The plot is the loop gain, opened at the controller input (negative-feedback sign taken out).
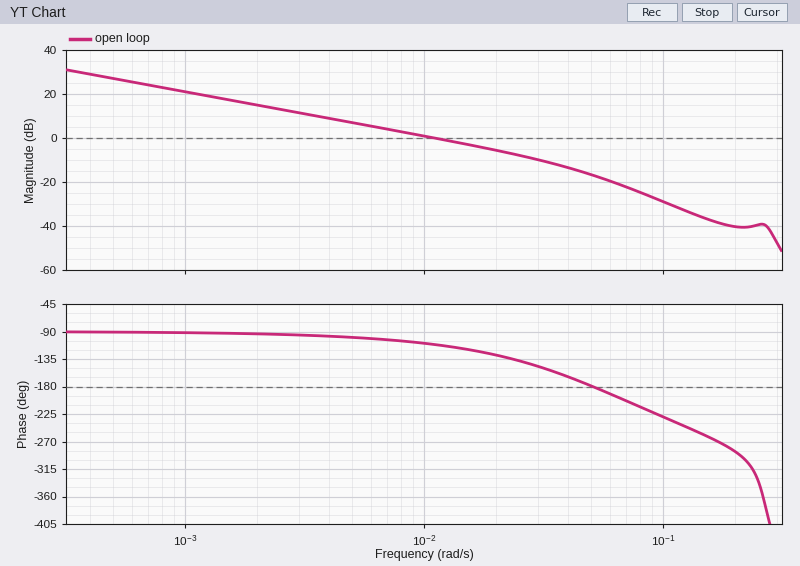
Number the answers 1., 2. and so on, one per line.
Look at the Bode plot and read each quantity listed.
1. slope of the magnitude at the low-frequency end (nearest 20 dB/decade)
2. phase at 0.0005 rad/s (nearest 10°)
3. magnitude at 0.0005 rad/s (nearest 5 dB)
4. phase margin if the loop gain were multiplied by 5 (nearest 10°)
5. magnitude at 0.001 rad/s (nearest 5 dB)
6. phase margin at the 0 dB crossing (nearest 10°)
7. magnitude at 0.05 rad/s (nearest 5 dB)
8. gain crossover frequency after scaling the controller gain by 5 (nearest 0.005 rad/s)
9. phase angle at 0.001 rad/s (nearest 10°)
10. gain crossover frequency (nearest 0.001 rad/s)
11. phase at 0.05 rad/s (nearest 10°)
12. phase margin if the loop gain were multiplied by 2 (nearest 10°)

1. -20 dB/decade
2. -90°
3. 25 dB
4. 10°
5. 20 dB
6. 70°
7. -15 dB
8. 0.040 rad/s
9. -90°
10. 0.011 rad/s
11. -180°
12. 50°
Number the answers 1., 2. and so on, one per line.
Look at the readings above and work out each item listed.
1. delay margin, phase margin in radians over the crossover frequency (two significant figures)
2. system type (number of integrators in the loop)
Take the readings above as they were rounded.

1. 110 s
2. 1
